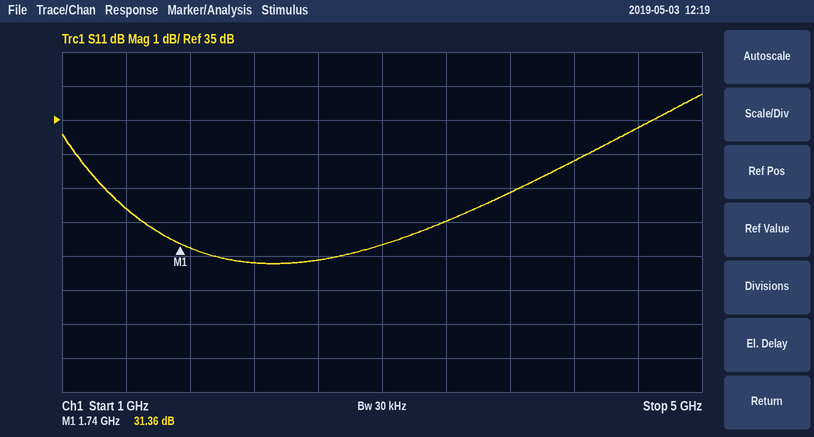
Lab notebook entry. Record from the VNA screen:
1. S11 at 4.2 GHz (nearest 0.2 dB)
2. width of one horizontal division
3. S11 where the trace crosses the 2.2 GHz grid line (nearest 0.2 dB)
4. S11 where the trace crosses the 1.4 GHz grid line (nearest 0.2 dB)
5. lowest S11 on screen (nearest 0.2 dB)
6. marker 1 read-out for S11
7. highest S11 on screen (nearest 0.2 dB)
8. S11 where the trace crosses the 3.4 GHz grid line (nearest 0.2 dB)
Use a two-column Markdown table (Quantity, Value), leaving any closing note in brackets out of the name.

| Quantity | Value |
|---|---|
| S11 at 4.2 GHz | 33.8 dB |
| width of one horizontal division | 400 MHz |
| S11 where the trace crosses the 2.2 GHz grid line | 30.8 dB |
| S11 where the trace crosses the 1.4 GHz grid line | 32.4 dB |
| lowest S11 on screen | 30.8 dB |
| marker 1 read-out for S11 | 31.36 dB |
| highest S11 on screen | 35.8 dB |
| S11 where the trace crosses the 3.4 GHz grid line | 32.0 dB |
